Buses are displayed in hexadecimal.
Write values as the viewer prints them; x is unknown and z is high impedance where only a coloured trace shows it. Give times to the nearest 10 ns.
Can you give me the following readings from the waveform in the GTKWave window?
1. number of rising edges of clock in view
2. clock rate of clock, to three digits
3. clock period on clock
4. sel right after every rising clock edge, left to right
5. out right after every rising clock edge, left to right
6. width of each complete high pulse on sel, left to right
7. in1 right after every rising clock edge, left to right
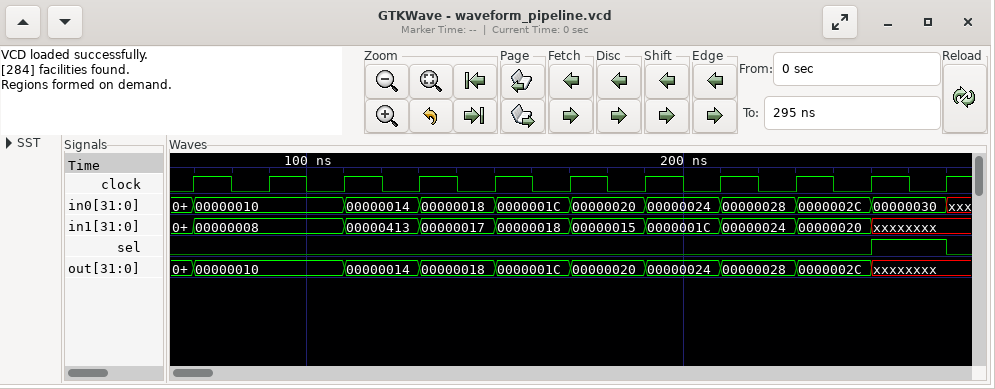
11
50.0 MHz
20 ns
0 0 0 0 0 0 0 0 0 1 0
00000010, 00000010, 00000014, 00000018, 0000001C, 00000020, 00000024, 00000028, 0000002C, xxxxxxxx, xxxxxxxx
20 ns
00000008, 00000008, 00000413, 00000017, 00000018, 00000015, 0000001C, 00000024, 00000020, xxxxxxxx, xxxxxxxx
